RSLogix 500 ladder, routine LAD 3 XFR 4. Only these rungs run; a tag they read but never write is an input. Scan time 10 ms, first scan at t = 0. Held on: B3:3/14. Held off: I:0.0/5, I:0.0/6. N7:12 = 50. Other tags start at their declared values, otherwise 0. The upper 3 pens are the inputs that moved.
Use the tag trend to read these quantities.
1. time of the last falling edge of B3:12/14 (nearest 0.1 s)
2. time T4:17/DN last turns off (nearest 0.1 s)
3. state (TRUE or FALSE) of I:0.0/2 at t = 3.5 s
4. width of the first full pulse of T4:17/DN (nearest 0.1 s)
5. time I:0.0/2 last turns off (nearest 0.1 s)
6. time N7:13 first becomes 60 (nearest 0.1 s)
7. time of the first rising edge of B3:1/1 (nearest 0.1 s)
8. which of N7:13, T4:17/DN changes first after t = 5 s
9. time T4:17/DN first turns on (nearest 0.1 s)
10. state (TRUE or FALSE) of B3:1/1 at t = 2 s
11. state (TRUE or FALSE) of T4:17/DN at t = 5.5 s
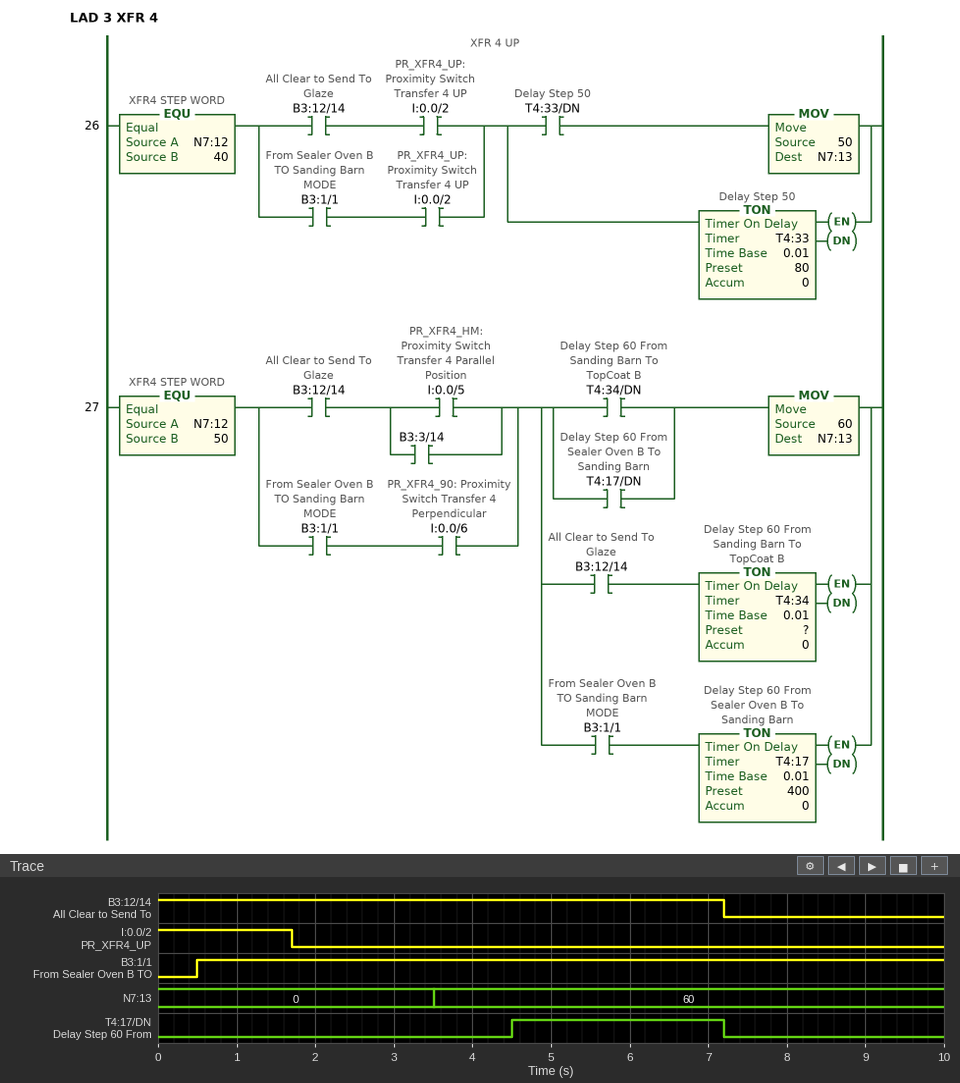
7.2 s
7.2 s
FALSE
2.7 s
1.7 s
3.5 s
0.5 s
T4:17/DN
4.5 s
TRUE
TRUE
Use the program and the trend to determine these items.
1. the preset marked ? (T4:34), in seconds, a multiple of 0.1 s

3.5 s
